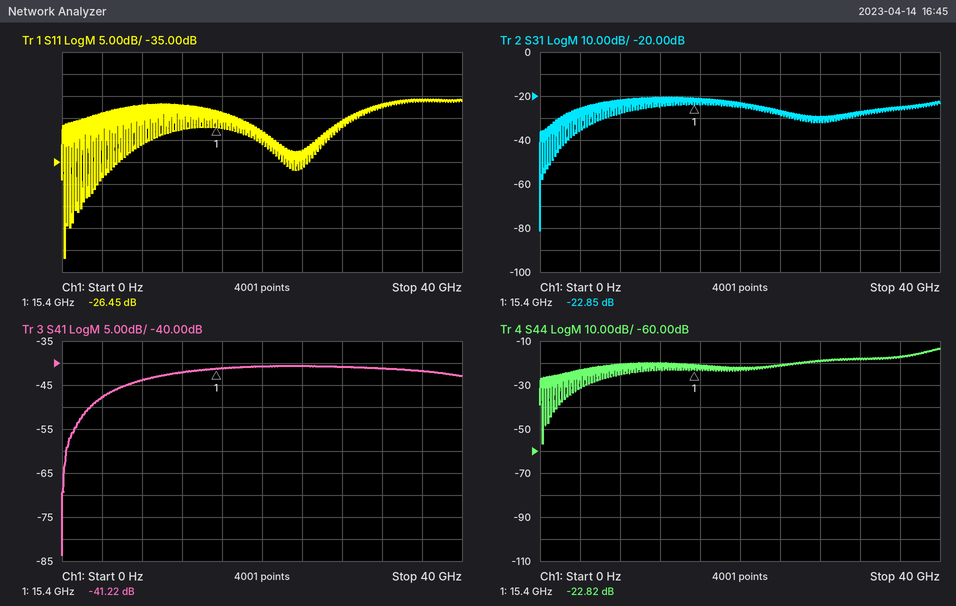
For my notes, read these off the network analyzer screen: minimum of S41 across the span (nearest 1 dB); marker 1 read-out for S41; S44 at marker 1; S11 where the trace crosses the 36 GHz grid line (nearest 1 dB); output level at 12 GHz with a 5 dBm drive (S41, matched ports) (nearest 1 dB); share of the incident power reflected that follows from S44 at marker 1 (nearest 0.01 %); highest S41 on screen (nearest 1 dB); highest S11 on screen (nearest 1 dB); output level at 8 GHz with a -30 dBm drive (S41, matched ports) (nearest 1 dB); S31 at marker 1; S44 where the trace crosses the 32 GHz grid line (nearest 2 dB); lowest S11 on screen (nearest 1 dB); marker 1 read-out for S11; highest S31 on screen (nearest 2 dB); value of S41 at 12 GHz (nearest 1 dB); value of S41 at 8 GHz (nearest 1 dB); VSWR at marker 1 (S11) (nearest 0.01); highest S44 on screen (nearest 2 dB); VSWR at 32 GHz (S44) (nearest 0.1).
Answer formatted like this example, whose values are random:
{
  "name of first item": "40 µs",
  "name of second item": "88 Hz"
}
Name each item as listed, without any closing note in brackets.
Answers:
{
  "minimum of S41 across the span": "-84 dB",
  "marker 1 read-out for S41": "-41.22 dB",
  "S44 at marker 1": "-22.82 dB",
  "S11 where the trace crosses the 36 GHz grid line": "-21 dB",
  "output level at 12 GHz with a 5 dBm drive (S41, matched ports)": "-37 dBm",
  "share of the incident power reflected that follows from S44 at marker 1": "0.52 %",
  "highest S41 on screen": "-41 dB",
  "highest S11 on screen": "-21 dB",
  "output level at 8 GHz with a -30 dBm drive (S41, matched ports)": "-74 dBm",
  "S31 at marker 1": "-22.85 dB",
  "S44 where the trace crosses the 32 GHz grid line": "-18 dB",
  "lowest S11 on screen": "-57 dB",
  "marker 1 read-out for S11": "-26.45 dB",
  "highest S31 on screen": "-20 dB",
  "value of S41 at 12 GHz": "-42 dB",
  "value of S41 at 8 GHz": "-44 dB",
  "VSWR at marker 1 (S11)": "1.10",
  "highest S44 on screen": "-14 dB",
  "VSWR at 32 GHz (S44)": "1.3"
}
